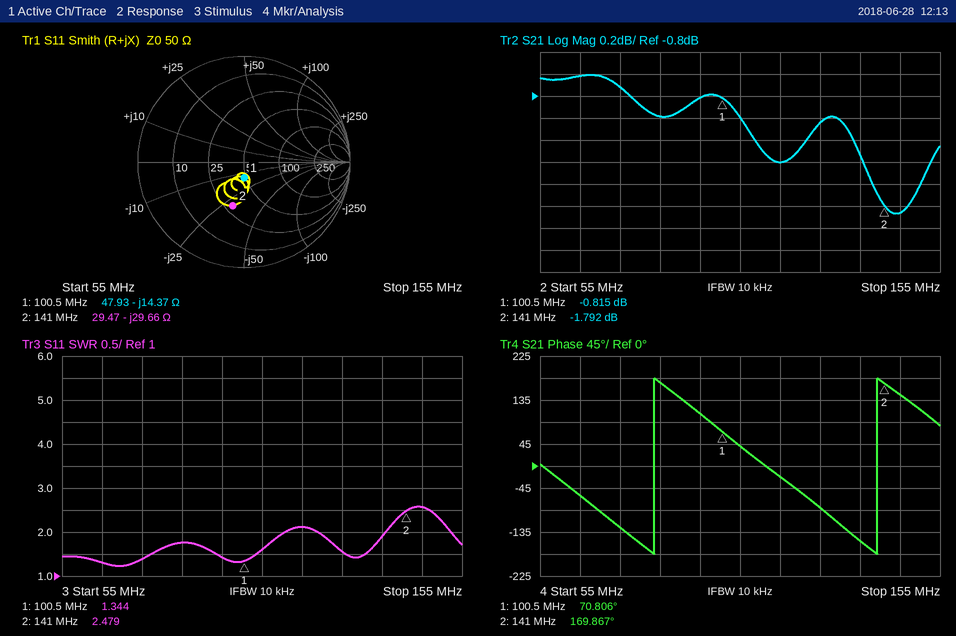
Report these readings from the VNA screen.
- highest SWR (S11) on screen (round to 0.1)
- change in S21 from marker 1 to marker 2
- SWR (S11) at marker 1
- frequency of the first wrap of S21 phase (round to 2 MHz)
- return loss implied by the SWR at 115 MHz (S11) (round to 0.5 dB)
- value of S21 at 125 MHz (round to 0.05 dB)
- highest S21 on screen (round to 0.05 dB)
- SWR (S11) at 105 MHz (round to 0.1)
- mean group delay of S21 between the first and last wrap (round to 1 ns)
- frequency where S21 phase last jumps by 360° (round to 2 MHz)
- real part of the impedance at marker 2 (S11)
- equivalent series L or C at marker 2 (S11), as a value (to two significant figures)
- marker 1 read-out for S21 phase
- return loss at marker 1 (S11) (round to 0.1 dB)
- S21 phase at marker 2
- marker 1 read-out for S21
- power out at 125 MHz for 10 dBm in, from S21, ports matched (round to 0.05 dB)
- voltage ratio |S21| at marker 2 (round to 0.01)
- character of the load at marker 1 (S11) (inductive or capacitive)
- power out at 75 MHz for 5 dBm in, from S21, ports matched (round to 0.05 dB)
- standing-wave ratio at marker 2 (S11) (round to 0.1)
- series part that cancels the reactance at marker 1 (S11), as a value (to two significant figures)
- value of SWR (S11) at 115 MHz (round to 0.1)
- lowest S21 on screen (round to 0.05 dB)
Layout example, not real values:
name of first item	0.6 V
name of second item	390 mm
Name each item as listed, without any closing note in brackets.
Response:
highest SWR (S11) on screen	2.6
change in S21 from marker 1 to marker 2	-0.977 dB
SWR (S11) at marker 1	1.344
frequency of the first wrap of S21 phase	84 MHz
return loss implied by the SWR at 115 MHz (S11)	9.0 dB
value of S21 at 125 MHz	-1.05 dB
highest S21 on screen	-0.60 dB
SWR (S11) at 105 MHz	1.6
mean group delay of S21 between the first and last wrap	18 ns
frequency where S21 phase last jumps by 360°	140 MHz
real part of the impedance at marker 2	29.47 Ω
equivalent series L or C at marker 2 (S11), as a value	38 pF
marker 1 read-out for S21 phase	70.806°
return loss at marker 1 (S11)	16.7 dB
S21 phase at marker 2	169.867°
marker 1 read-out for S21	-0.815 dB
power out at 125 MHz for 10 dBm in, from S21, ports matched	8.95 dBm
voltage ratio |S21| at marker 2	0.81
character of the load at marker 1 (S11)	capacitive
power out at 75 MHz for 5 dBm in, from S21, ports matched	4.30 dBm
standing-wave ratio at marker 2 (S11)	2.5
series part that cancels the reactance at marker 1 (S11), as a value	23 nH
value of SWR (S11) at 115 MHz	2.1
lowest S21 on screen	-1.85 dB
